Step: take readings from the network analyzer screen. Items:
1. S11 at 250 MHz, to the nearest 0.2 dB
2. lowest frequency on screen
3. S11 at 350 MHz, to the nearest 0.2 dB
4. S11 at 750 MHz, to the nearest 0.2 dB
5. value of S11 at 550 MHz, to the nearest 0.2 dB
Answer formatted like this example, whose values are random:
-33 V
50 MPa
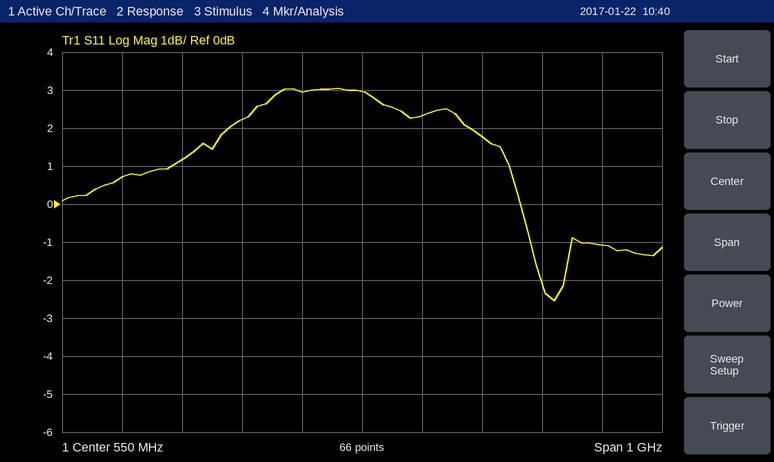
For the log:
1.2 dB
50 MHz
2.2 dB
1.8 dB
3.0 dB
